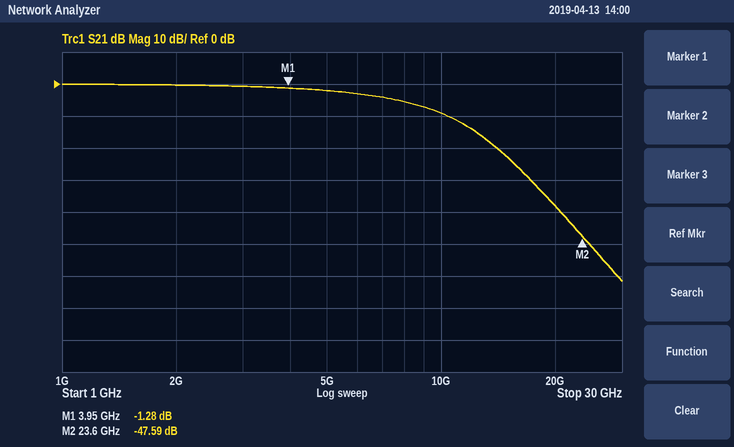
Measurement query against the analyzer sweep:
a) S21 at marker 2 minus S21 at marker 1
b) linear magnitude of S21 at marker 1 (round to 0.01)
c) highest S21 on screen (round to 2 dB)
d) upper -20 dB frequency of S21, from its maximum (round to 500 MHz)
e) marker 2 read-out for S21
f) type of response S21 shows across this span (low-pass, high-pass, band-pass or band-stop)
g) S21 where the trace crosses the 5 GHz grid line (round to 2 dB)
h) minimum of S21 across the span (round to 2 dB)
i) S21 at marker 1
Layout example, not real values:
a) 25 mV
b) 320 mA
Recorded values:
a) -46.31 dB
b) 0.86
c) 0 dB
d) 14.0 GHz
e) -47.59 dB
f) low-pass
g) -2 dB
h) -62 dB
i) -1.28 dB
